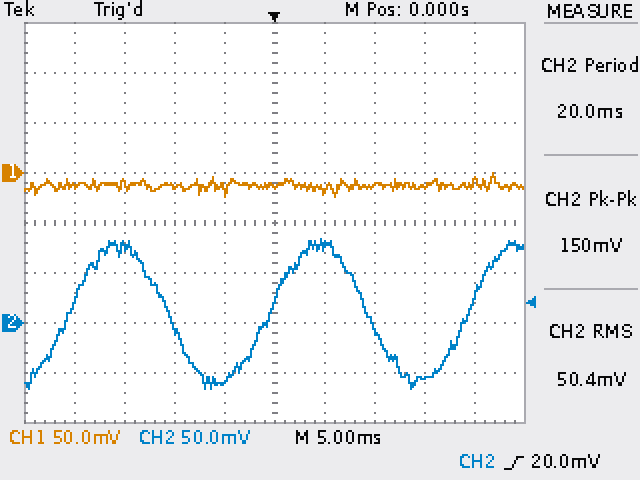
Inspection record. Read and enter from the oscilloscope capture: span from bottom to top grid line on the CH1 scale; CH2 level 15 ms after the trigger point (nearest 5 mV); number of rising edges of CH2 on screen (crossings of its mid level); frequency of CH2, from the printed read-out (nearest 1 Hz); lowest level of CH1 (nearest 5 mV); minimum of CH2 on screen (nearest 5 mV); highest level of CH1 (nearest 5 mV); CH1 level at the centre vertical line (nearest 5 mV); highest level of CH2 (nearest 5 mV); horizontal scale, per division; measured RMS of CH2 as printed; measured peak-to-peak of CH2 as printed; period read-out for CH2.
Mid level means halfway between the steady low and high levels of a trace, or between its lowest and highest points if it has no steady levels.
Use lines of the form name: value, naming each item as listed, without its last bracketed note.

span from bottom to top grid line on the CH1 scale: 400 mV
CH2 level 15 ms after the trigger point: -55 mV
number of rising edges of CH2 on screen: 3
frequency of CH2, from the printed read-out: 50 Hz
lowest level of CH1: -25 mV
minimum of CH2 on screen: -65 mV
highest level of CH1: 0 mV
CH1 level at the centre vertical line: -15 mV
highest level of CH2: 85 mV
horizontal scale, per division: 5 ms
measured RMS of CH2 as printed: 50.4 mV
measured peak-to-peak of CH2 as printed: 150 mV
period read-out for CH2: 20.0 ms
